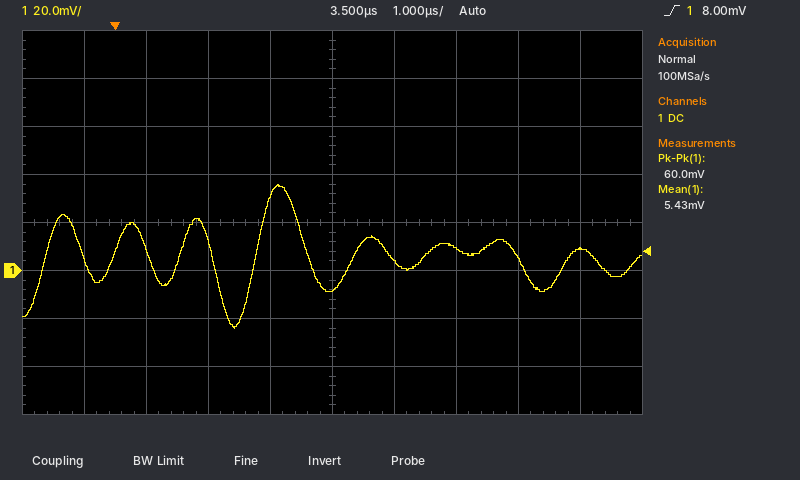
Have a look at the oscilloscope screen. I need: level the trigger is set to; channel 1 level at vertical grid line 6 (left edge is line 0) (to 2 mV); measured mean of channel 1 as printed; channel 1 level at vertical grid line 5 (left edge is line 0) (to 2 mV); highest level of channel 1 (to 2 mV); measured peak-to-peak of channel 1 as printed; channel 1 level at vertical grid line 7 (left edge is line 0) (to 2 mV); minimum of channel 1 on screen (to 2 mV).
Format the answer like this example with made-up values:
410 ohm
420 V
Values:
8.00 mV
4 mV
5.43 mV
-8 mV
36 mV
60.0 mV
10 mV
-24 mV
